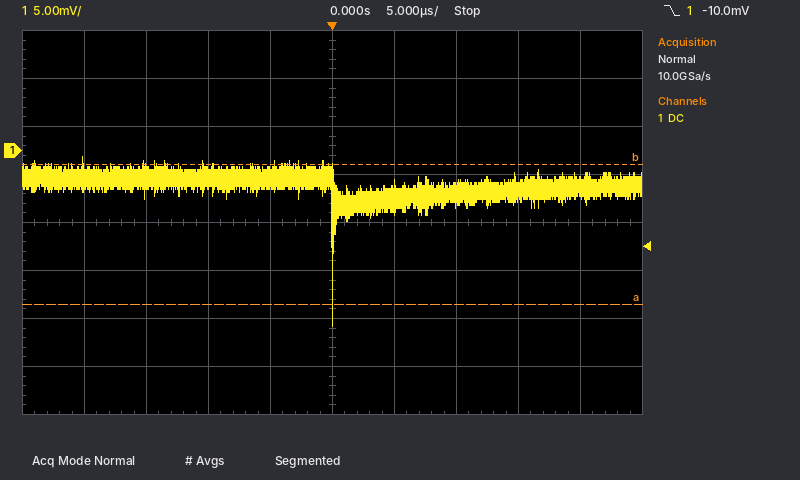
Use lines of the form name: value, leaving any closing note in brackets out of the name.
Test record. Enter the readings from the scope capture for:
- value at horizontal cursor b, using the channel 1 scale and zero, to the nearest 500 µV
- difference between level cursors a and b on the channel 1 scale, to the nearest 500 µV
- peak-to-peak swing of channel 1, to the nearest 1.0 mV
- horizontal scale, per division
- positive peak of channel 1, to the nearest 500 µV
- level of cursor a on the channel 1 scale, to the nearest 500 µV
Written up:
value at horizontal cursor b, using the channel 1 scale and zero, to the nearest 500 µV: -1.5 mV
difference between level cursors a and b on the channel 1 scale, to the nearest 500 µV: 14.5 mV
peak-to-peak swing of channel 1, to the nearest 1.0 mV: 18.0 mV
horizontal scale, per division: 5 µs
positive peak of channel 1, to the nearest 500 µV: -500 µV
level of cursor a on the channel 1 scale, to the nearest 500 µV: -16.0 mV
